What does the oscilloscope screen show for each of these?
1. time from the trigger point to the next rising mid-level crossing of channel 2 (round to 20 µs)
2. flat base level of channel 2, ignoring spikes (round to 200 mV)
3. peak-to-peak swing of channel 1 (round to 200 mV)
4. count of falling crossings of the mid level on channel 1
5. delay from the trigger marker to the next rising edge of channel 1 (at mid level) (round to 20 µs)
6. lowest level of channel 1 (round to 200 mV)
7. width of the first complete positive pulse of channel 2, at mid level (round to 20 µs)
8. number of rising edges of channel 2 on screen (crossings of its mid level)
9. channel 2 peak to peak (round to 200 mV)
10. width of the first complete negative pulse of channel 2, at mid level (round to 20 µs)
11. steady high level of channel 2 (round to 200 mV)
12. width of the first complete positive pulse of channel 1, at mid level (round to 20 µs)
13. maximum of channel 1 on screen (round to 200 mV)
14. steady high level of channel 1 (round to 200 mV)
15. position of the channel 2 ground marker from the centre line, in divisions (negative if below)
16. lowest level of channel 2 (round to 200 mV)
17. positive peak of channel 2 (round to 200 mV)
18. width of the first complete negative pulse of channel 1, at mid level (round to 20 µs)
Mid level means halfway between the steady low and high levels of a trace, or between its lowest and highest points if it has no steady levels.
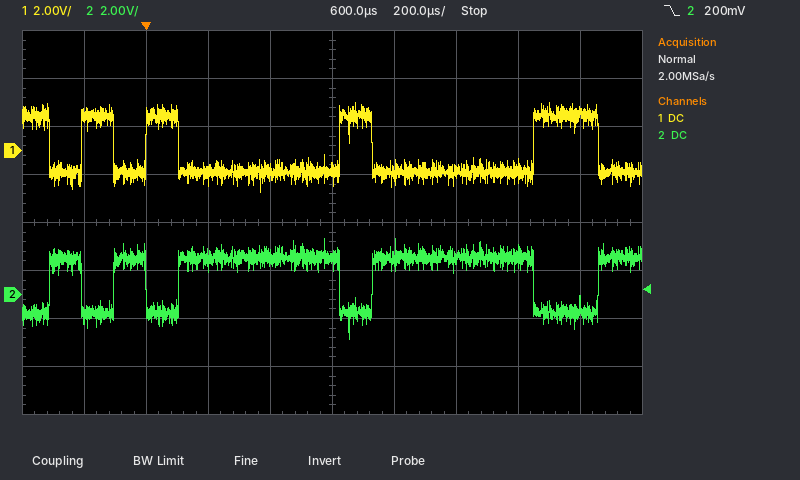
100 µs
-800 mV
3.8 V
5
620 µs
-1.8 V
100 µs
5
4.2 V
100 µs
1.6 V
100 µs
2.0 V
1.4 V
-1.5 div
-1.8 V
2.4 V
100 µs
